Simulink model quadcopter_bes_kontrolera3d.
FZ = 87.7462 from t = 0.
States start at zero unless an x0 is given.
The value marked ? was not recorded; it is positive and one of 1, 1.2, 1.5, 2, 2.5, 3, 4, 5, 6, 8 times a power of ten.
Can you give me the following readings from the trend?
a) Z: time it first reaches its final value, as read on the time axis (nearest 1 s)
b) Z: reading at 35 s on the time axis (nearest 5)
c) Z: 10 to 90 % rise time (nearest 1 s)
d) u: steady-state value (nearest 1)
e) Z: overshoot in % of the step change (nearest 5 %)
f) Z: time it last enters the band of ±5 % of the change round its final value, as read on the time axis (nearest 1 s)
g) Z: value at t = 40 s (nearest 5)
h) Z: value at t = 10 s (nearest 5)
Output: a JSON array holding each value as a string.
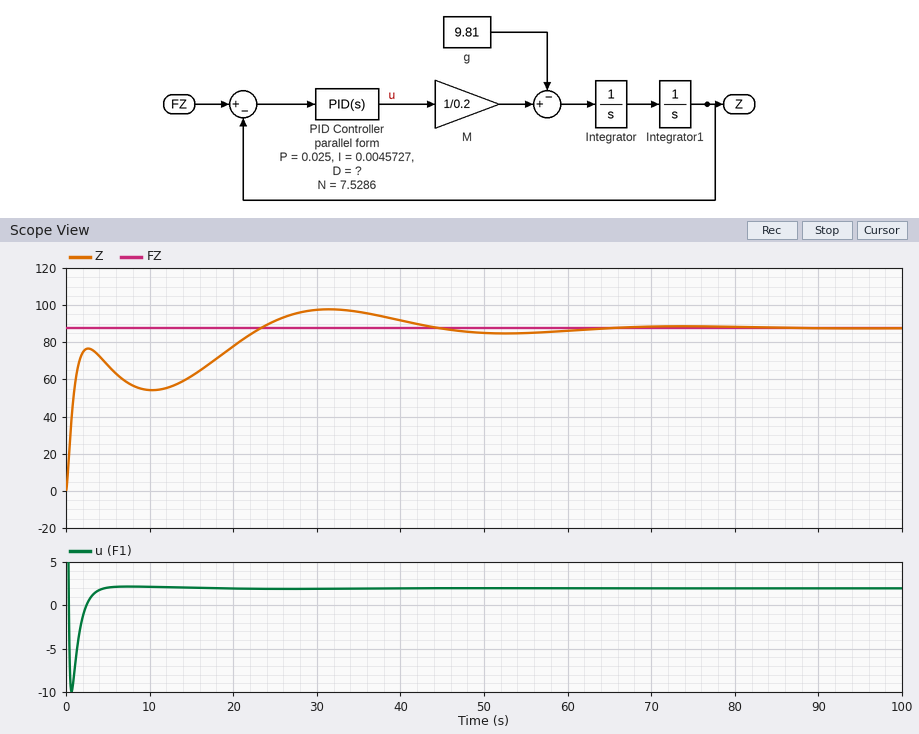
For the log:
["23 s", "95", "20 s", "2", "10 %", "40 s", "90", "55"]
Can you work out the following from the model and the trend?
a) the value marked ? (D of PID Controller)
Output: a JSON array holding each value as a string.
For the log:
["0.2"]
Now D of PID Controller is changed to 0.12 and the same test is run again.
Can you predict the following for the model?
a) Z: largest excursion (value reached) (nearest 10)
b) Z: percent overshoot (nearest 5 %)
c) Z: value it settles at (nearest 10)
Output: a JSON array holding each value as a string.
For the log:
["100", "10 %", "90"]
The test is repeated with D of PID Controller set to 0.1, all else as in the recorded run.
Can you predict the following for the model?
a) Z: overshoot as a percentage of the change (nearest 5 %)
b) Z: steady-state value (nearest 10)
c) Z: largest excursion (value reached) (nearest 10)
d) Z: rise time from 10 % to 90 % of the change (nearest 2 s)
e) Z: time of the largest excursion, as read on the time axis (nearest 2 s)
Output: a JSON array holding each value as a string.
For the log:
["10 %", "90", "100", "16 s", "24 s"]
